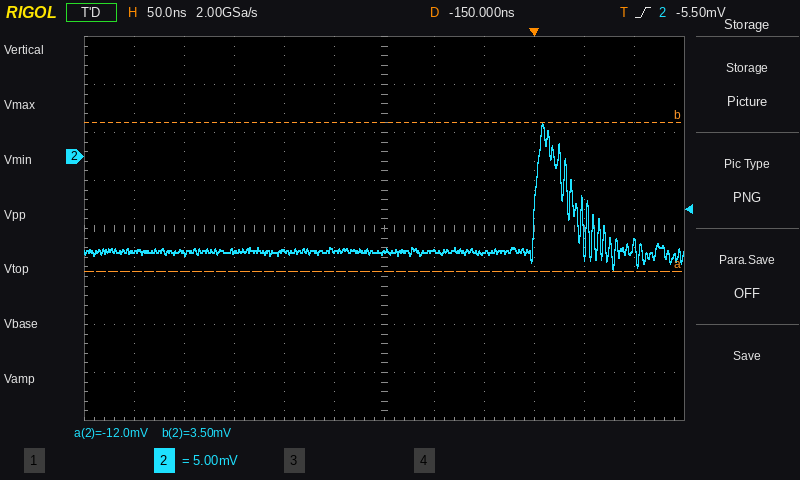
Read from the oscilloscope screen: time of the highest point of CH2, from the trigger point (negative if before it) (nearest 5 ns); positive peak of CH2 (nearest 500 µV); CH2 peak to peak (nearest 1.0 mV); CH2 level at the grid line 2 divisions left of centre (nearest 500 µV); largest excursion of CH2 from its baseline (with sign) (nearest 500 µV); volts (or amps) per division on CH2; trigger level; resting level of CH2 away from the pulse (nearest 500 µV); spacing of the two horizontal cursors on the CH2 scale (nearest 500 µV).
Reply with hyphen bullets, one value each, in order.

- +10 ns
- 3.5 mV
- 15.0 mV
- -10.0 mV
- +13.5 mV
- 5 mV
- -5.50 mV
- -10.0 mV
- 15.5 mV
